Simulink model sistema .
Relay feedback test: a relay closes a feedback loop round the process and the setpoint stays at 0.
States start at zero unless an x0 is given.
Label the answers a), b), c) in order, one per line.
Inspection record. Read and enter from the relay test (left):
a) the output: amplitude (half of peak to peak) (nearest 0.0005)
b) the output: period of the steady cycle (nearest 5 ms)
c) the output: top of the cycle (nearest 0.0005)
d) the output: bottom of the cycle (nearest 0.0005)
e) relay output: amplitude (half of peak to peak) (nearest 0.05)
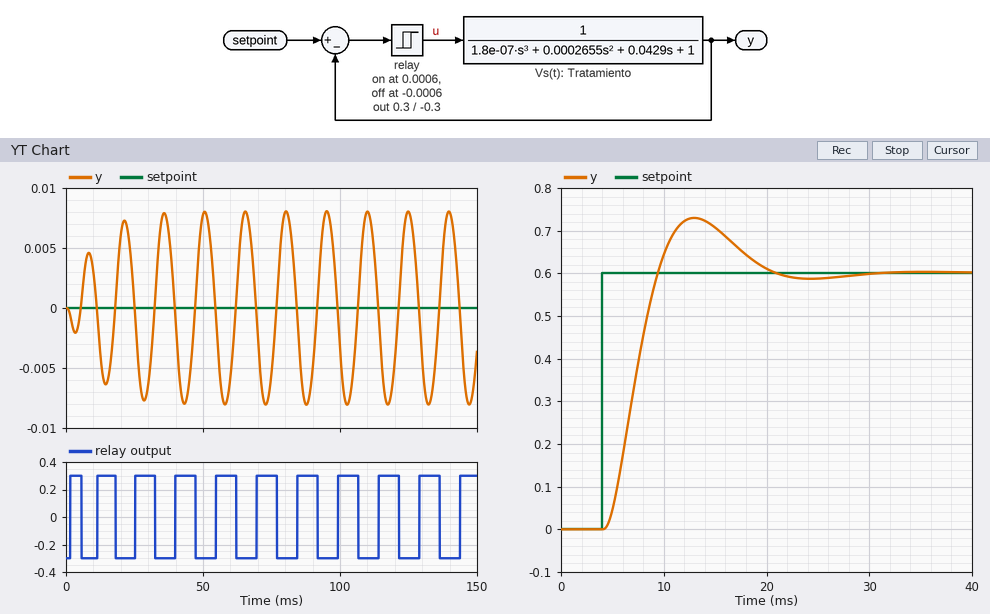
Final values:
a) 0.0080
b) 15 ms
c) 0.0080
d) -0.0080
e) 0.30
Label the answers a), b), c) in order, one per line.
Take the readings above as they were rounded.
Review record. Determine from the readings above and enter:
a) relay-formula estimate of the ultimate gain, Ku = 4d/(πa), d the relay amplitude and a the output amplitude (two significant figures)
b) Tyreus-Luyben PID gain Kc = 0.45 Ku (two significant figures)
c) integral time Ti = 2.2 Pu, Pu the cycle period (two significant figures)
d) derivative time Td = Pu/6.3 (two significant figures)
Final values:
a) 48
b) 22
c) 33 ms
d) 2.4 ms
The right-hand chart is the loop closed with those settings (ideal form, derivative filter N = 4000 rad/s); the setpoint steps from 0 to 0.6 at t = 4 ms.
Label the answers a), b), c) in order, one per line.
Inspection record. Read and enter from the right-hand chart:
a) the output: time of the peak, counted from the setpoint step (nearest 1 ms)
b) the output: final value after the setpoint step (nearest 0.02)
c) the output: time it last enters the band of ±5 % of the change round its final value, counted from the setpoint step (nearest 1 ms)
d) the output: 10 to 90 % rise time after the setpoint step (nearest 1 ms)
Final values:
a) 9 ms
b) 0.60
c) 15 ms
d) 4 ms
